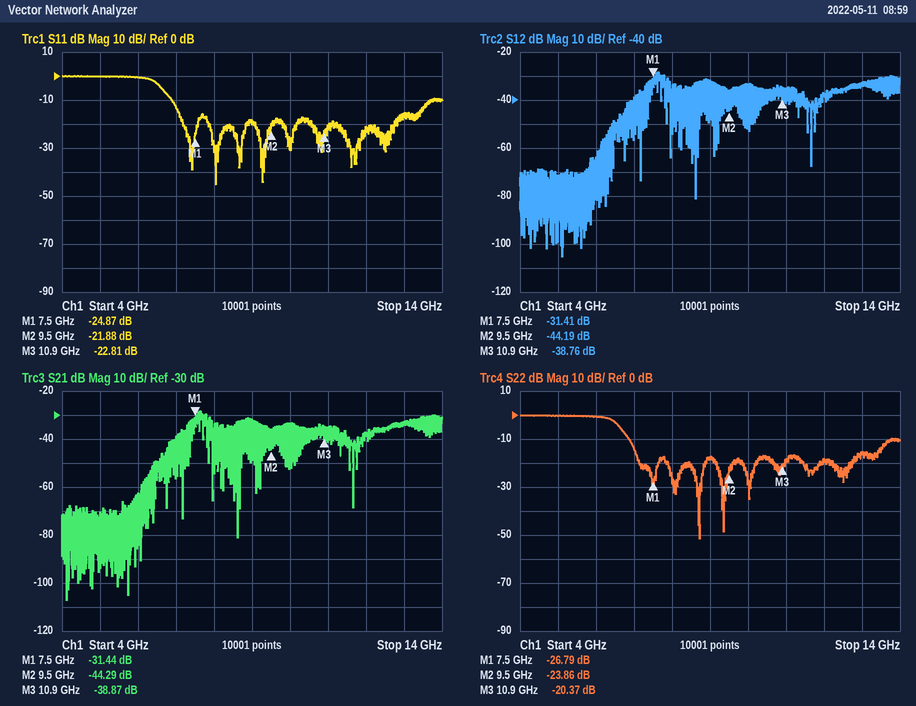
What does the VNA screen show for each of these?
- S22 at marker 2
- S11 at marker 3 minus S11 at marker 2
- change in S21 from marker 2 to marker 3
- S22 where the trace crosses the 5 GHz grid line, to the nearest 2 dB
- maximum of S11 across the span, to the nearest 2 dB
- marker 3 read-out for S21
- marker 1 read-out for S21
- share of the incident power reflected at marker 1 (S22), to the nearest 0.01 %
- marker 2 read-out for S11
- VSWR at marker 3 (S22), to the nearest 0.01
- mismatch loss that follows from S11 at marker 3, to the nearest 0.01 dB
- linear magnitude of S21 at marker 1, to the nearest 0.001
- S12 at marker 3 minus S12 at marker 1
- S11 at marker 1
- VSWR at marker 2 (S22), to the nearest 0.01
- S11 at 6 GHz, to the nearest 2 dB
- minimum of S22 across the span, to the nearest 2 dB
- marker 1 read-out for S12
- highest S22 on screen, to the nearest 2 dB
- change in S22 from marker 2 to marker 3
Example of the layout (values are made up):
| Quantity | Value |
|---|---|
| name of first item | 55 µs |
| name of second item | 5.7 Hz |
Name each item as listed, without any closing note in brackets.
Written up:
| Quantity | Value |
|---|---|
| S22 at marker 2 | -23.86 dB |
| S11 at marker 3 minus S11 at marker 2 | -0.93 dB |
| change in S21 from marker 2 to marker 3 | 5.42 dB |
| S22 where the trace crosses the 5 GHz grid line, to the nearest 2 dB | 0 dB |
| maximum of S11 across the span, to the nearest 2 dB | 0 dB |
| marker 3 read-out for S21 | -38.87 dB |
| marker 1 read-out for S21 | -31.44 dB |
| share of the incident power reflected at marker 1 (S22), to the nearest 0.01 % | 0.21 % |
| marker 2 read-out for S11 | -21.88 dB |
| VSWR at marker 3 (S22), to the nearest 0.01 | 1.21 |
| mismatch loss that follows from S11 at marker 3, to the nearest 0.01 dB | 0.02 dB |
| linear magnitude of S21 at marker 1, to the nearest 0.001 | 0.027 |
| S12 at marker 3 minus S12 at marker 1 | -7.35 dB |
| S11 at marker 1 | -24.87 dB |
| VSWR at marker 2 (S22), to the nearest 0.01 | 1.14 |
| S11 at 6 GHz, to the nearest 2 dB | 0 dB |
| minimum of S22 across the span, to the nearest 2 dB | -52 dB |
| marker 1 read-out for S12 | -31.41 dB |
| highest S22 on screen, to the nearest 2 dB | 0 dB |
| change in S22 from marker 2 to marker 3 | 3.49 dB |
